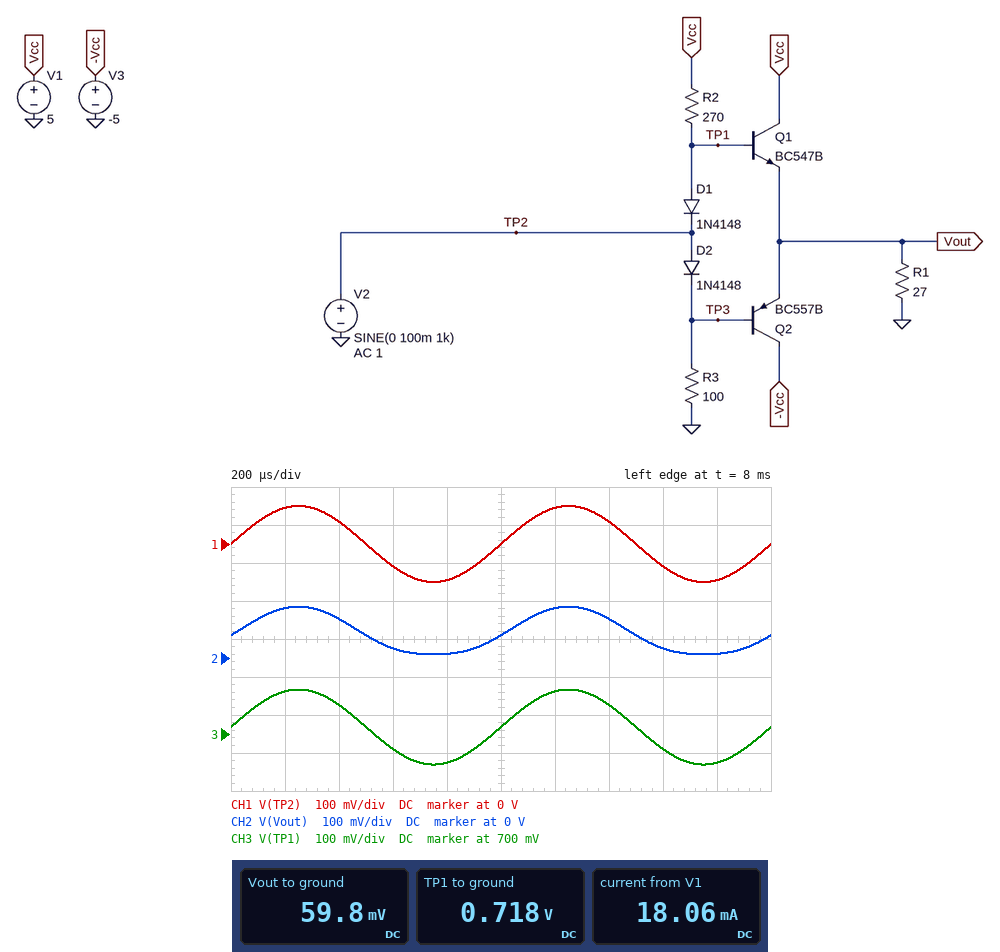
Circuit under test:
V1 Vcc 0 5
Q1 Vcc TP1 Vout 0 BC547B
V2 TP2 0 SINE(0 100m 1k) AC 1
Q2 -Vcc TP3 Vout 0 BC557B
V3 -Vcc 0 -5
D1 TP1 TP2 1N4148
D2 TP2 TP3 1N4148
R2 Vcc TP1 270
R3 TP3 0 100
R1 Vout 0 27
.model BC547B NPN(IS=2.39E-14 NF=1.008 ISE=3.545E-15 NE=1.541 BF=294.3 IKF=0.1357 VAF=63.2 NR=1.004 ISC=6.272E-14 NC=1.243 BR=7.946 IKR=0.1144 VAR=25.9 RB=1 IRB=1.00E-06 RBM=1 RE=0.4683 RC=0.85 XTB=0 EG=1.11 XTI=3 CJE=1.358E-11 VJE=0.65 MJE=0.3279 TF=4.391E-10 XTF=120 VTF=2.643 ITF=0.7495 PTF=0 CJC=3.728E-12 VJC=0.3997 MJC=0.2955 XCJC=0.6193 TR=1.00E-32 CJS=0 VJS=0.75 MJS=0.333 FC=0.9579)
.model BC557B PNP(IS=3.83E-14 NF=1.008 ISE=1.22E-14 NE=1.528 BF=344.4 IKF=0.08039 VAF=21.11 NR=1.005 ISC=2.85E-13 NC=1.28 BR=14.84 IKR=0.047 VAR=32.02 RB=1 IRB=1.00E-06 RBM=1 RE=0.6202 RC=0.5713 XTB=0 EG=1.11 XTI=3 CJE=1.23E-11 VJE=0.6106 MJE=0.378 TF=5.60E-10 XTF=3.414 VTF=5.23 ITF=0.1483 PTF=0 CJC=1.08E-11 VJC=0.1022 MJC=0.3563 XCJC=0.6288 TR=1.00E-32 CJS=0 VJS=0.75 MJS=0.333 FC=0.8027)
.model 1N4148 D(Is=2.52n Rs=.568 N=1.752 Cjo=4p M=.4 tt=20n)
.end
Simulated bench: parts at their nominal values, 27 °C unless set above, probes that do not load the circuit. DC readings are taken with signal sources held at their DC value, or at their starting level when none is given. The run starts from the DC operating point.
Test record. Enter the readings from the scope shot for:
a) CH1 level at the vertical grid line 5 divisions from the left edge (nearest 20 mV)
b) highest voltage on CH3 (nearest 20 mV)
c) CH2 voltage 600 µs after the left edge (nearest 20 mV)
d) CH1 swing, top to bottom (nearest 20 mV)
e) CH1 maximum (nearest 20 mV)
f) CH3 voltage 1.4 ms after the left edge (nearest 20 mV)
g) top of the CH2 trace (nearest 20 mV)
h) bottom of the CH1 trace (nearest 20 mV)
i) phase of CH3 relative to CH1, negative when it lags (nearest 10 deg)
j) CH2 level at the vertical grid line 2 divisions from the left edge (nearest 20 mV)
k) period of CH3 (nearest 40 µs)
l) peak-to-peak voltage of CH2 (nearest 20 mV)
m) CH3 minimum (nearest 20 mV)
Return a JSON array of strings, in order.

["0 V", "820 mV", "20 mV", "200 mV", "100 mV", "780 mV", "140 mV", "-100 mV", "0 deg", "100 mV", "1.00 ms", "120 mV", "620 mV"]
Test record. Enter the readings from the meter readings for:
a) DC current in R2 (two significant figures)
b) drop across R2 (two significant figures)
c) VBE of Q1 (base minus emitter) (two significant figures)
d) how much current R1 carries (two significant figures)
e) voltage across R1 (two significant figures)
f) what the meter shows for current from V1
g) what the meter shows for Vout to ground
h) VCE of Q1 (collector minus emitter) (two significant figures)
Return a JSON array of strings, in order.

["16 mA", "4.3 V", "660 mV", "2.2 mA", "60 mV", "18.06 mA", "59.8 mV", "4.9 V"]
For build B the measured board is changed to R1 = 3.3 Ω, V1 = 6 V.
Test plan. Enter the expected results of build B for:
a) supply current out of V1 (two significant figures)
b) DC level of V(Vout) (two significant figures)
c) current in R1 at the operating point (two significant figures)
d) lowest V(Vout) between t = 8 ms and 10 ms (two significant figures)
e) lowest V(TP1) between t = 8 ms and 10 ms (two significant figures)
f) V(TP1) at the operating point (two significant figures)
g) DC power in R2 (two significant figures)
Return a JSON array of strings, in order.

["29 mA", "30 mV", "9.1 mA", "2.4 mV", "630 mV", "730 mV", "100 mW"]
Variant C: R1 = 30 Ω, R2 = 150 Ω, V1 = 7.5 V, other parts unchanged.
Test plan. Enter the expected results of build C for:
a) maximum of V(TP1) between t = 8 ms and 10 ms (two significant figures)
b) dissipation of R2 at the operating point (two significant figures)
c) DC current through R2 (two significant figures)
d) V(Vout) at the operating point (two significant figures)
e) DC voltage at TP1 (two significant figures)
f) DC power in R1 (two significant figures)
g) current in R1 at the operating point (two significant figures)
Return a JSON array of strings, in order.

["880 mV", "300 mW", "45 mA", "110 mV", "780 mV", "400 µW", "3.7 mA"]
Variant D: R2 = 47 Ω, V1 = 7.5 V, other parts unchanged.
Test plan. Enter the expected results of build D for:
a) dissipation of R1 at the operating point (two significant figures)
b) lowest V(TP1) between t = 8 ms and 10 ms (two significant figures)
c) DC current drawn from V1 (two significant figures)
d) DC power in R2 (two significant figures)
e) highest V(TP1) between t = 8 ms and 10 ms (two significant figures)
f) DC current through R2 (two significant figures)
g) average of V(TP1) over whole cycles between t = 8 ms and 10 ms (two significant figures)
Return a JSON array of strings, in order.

["1.4 mW", "790 mV", "150 mA", "930 mW", "990 mV", "140 mA", "890 mV"]
